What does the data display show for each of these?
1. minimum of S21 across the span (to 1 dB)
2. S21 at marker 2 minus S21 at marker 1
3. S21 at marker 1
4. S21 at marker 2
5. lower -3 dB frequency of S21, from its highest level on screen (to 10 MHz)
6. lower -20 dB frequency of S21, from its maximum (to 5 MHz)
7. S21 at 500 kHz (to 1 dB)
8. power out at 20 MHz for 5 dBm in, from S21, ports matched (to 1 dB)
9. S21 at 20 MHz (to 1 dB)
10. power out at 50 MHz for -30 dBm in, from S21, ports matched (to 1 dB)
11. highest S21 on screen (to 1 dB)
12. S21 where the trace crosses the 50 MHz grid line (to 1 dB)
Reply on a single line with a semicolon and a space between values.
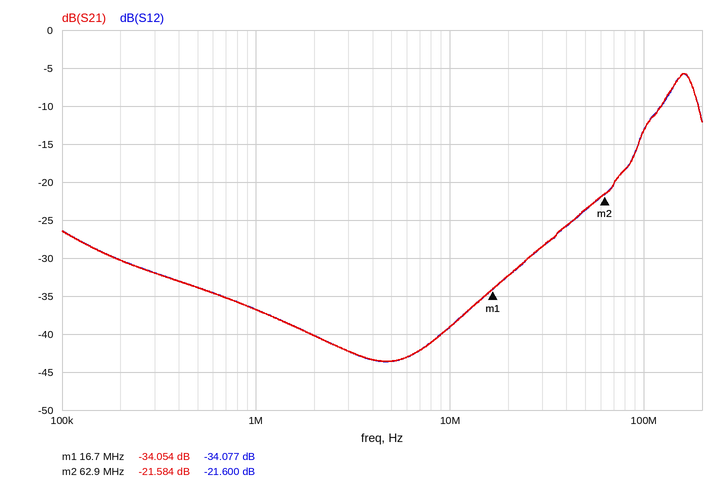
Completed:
-44 dB; 12.470 dB; -34.054 dB; -21.584 dB; 130 MHz; 40 MHz; -34 dB; -27 dBm; -32 dB; -54 dBm; -6 dB; -24 dB
